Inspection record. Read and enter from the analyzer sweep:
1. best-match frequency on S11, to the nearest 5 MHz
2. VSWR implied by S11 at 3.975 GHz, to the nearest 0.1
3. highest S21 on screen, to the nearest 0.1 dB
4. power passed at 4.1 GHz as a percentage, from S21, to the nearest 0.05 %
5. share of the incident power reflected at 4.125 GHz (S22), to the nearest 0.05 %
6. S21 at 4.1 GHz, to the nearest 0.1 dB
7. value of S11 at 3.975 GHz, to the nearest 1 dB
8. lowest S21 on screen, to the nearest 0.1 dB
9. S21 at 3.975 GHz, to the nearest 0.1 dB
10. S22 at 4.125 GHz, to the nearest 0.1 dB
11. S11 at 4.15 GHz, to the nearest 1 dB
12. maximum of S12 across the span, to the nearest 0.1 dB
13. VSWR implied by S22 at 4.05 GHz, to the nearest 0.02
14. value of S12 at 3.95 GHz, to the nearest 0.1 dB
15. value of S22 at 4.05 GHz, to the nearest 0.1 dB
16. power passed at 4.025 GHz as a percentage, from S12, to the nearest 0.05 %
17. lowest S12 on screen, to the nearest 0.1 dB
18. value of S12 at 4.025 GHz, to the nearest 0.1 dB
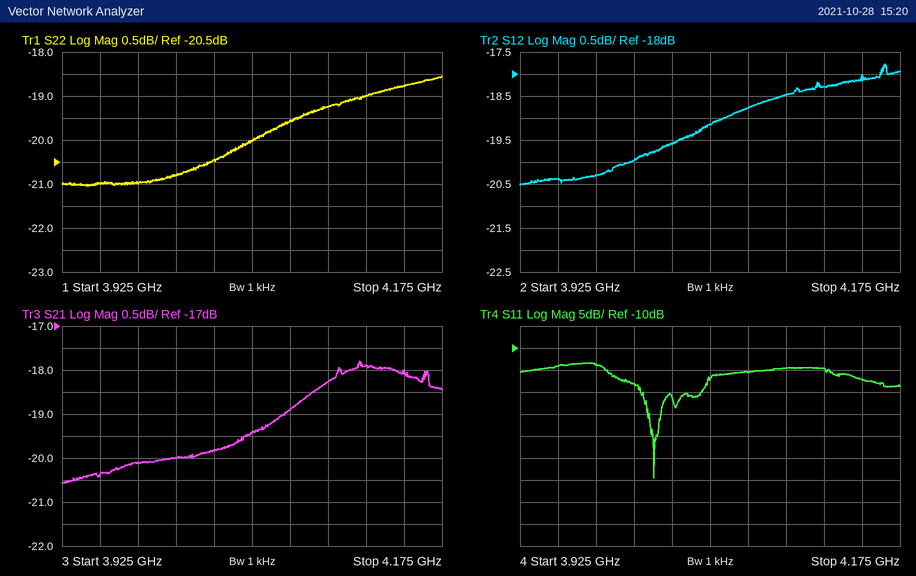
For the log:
4.015 GHz
1.5
-17.8 dB
1.50 %
1.25 %
-18.3 dB
-14 dB
-20.6 dB
-20.1 dB
-19.0 dB
-17 dB
-17.8 dB
1.22
-20.4 dB
-20.0 dB
1.10 %
-20.5 dB
-19.6 dB
